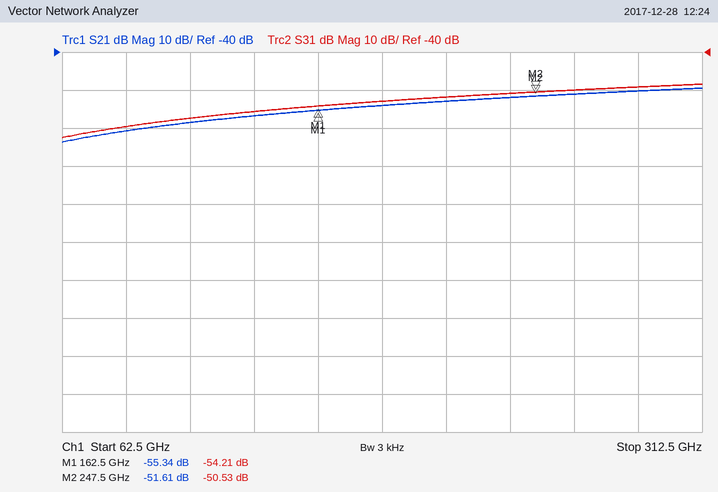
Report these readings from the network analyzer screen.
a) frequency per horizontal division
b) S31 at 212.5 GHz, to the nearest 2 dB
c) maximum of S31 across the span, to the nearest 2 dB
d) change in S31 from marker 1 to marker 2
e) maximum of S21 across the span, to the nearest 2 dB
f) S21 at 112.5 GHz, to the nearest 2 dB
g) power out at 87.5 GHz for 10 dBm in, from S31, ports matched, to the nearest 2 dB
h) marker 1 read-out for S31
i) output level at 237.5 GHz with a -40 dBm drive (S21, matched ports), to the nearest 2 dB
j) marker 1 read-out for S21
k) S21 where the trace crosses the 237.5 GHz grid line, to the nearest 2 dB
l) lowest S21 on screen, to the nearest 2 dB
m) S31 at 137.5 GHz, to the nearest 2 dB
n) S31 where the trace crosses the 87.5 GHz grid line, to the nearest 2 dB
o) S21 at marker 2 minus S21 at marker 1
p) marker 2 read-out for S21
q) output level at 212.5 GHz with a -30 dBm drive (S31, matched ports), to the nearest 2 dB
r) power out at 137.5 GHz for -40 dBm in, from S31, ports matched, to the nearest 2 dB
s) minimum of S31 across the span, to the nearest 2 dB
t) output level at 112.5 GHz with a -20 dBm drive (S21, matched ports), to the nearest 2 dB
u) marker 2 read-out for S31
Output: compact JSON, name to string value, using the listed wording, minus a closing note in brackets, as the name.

{"frequency per horizontal division": "25 GHz", "S31 at 212.5 GHz, to the nearest 2 dB": "-52 dB", "maximum of S31 across the span, to the nearest 2 dB": "-48 dB", "change in S31 from marker 1 to marker 2": "3.68 dB", "maximum of S21 across the span, to the nearest 2 dB": "-50 dB", "S21 at 112.5 GHz, to the nearest 2 dB": "-58 dB", "power out at 87.5 GHz for 10 dBm in, from S31, ports matched, to the nearest 2 dB": "-50 dBm", "marker 1 read-out for S31": "-54.21 dB", "output level at 237.5 GHz with a -40 dBm drive (S21, matched ports), to the nearest 2 dB": "-92 dBm", "marker 1 read-out for S21": "-55.34 dB", "S21 where the trace crosses the 237.5 GHz grid line, to the nearest 2 dB": "-52 dB", "lowest S21 on screen, to the nearest 2 dB": "-64 dB", "S31 at 137.5 GHz, to the nearest 2 dB": "-56 dB", "S31 where the trace crosses the 87.5 GHz grid line, to the nearest 2 dB": "-60 dB", "S21 at marker 2 minus S21 at marker 1": "3.73 dB", "marker 2 read-out for S21": "-51.61 dB", "output level at 212.5 GHz with a -30 dBm drive (S31, matched ports), to the nearest 2 dB": "-82 dBm", "power out at 137.5 GHz for -40 dBm in, from S31, ports matched, to the nearest 2 dB": "-96 dBm", "minimum of S31 across the span, to the nearest 2 dB": "-62 dB", "output level at 112.5 GHz with a -20 dBm drive (S21, matched ports), to the nearest 2 dB": "-78 dBm", "marker 2 read-out for S31": "-50.53 dB"}
